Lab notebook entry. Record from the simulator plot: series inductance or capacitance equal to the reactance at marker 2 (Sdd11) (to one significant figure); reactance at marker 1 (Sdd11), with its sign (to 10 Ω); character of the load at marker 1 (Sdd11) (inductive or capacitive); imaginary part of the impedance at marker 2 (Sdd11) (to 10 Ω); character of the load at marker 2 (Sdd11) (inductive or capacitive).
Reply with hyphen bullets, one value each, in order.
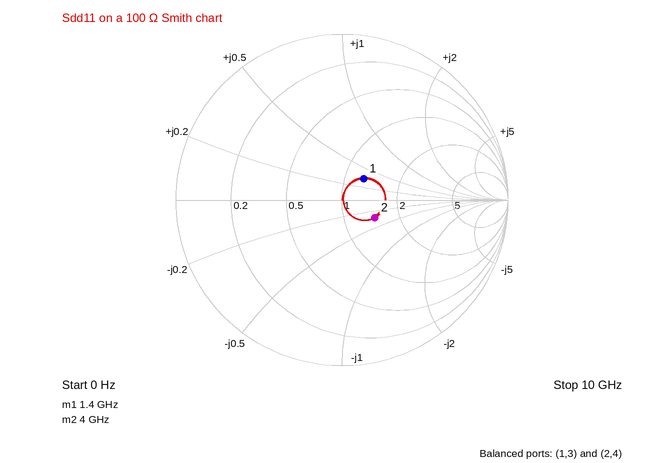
- 1 pF
- +30 Ω
- inductive
- -30 Ω
- capacitive
